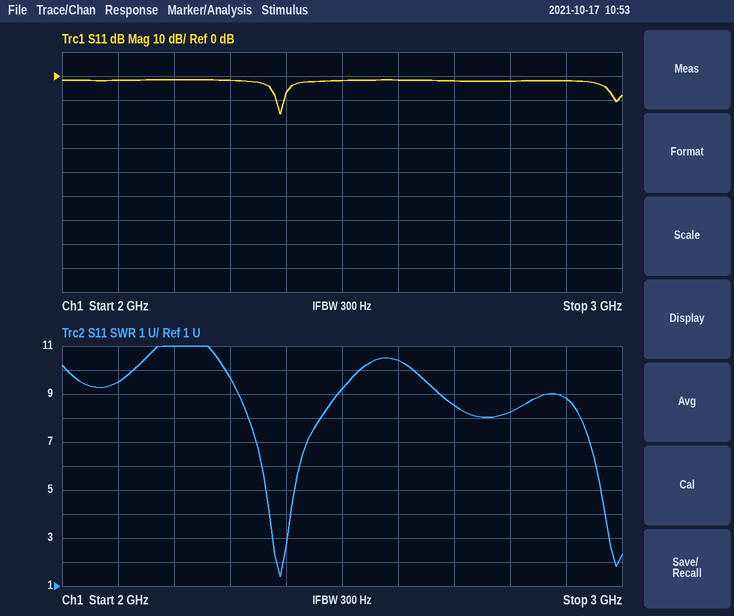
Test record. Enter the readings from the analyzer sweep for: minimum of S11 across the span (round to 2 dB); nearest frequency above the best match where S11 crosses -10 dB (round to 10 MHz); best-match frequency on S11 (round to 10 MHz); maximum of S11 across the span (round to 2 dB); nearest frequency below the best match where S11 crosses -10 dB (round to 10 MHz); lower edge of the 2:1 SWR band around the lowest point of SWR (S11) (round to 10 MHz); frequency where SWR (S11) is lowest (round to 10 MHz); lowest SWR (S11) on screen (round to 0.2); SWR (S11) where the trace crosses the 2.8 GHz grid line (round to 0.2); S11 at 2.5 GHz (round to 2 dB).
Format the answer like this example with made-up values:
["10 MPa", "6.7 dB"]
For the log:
["-16 dB", "2.40 GHz", "2.39 GHz", "-2 dB", "2.38 GHz", "2.38 GHz", "2.39 GHz", "1.4", "8.2", "-2 dB"]
